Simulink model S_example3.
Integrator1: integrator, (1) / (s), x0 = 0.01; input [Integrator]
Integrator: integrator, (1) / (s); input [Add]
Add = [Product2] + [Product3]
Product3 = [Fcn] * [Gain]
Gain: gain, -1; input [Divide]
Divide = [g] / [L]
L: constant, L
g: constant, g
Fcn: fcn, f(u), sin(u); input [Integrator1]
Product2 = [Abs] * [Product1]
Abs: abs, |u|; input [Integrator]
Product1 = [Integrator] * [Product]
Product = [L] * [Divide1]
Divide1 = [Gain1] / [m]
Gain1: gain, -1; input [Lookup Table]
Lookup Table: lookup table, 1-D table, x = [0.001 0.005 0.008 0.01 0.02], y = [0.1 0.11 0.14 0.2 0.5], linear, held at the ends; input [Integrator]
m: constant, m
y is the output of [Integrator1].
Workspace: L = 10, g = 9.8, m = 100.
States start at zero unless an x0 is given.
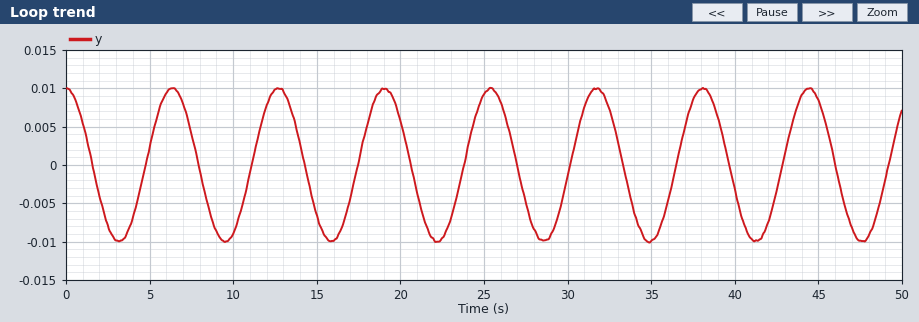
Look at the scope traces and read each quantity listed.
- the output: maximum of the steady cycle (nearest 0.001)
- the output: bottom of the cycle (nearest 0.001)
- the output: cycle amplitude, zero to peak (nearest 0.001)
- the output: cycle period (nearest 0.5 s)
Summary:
0.010
-0.010
0.010
6.5 s
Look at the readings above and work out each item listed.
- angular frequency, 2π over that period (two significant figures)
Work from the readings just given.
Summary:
0.97 rad/s
